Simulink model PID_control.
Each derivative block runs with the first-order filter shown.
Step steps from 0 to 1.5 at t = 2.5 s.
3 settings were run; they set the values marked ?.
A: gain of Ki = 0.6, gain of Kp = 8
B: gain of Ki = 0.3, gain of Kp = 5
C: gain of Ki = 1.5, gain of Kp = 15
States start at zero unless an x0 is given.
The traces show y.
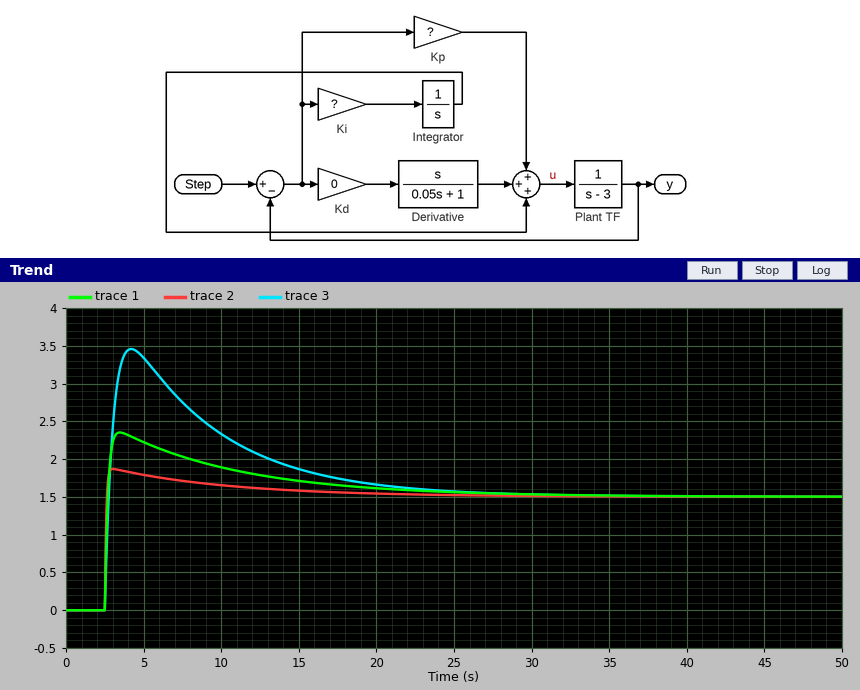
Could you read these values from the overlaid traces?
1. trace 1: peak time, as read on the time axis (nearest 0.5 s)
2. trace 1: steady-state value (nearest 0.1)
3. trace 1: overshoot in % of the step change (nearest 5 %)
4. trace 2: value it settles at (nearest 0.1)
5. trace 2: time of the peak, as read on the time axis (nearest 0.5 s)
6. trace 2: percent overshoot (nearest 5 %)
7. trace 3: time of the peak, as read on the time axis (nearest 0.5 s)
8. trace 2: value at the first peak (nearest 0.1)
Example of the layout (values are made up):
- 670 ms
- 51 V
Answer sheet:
- 3.5 s
- 1.5
- 55 %
- 1.5
- 3.0 s
- 25 %
- 4.0 s
- 1.9
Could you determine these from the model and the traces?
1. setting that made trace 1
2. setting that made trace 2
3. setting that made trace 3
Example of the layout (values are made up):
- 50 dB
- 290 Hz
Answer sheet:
- A
- C
- B
